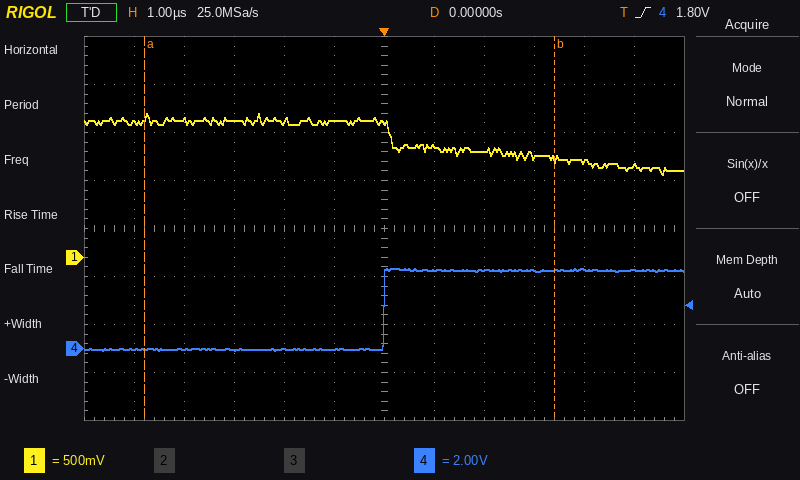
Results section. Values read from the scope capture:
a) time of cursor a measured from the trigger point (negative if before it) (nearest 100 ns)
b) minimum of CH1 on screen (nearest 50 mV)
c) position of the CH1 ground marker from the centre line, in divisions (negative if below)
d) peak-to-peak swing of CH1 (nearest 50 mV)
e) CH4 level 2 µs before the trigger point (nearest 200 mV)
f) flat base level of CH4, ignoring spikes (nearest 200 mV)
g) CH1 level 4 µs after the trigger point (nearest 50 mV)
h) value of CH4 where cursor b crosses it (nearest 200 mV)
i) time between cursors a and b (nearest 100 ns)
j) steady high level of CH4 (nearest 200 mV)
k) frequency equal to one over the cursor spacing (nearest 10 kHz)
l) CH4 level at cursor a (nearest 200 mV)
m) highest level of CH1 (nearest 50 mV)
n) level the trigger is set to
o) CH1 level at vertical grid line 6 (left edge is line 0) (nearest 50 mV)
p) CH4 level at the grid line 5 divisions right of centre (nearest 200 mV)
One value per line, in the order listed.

-4.8 µs
850 mV
-0.6 div
650 mV
0.0 V
0.0 V
1.00 V
3.2 V
8.2 µs
3.2 V
120 kHz
0.0 V
1.50 V
1.80 V
1.40 V
3.2 V
